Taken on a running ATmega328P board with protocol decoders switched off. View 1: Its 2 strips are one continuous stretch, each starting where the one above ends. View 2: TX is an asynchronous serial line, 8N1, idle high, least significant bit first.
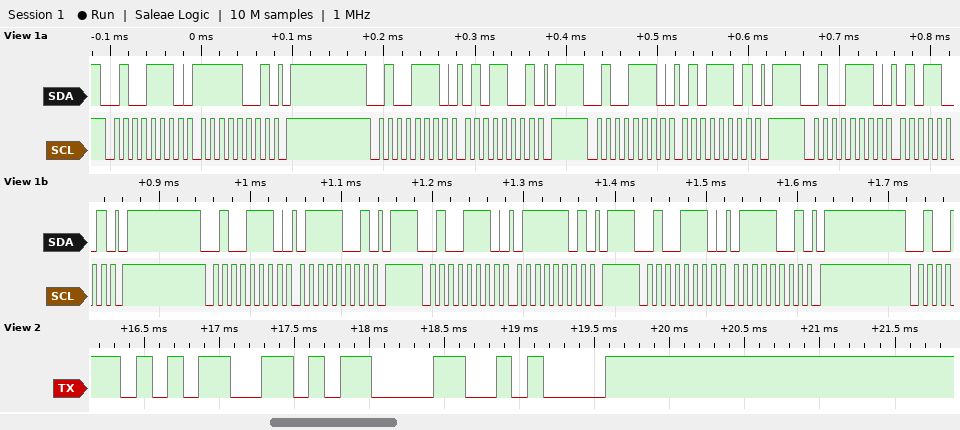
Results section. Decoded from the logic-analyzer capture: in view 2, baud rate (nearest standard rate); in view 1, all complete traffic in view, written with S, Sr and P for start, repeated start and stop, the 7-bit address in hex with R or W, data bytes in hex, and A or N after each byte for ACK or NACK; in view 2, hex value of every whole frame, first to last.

9600 baud
S 27W A F9 A P S 27W A 59 A P S 27W A 5D A P S 27W A 59 A P S 27W A 79 A P S 27W A 7D A P S 27W A 79 A P
0x35 0x0D 0x0A
